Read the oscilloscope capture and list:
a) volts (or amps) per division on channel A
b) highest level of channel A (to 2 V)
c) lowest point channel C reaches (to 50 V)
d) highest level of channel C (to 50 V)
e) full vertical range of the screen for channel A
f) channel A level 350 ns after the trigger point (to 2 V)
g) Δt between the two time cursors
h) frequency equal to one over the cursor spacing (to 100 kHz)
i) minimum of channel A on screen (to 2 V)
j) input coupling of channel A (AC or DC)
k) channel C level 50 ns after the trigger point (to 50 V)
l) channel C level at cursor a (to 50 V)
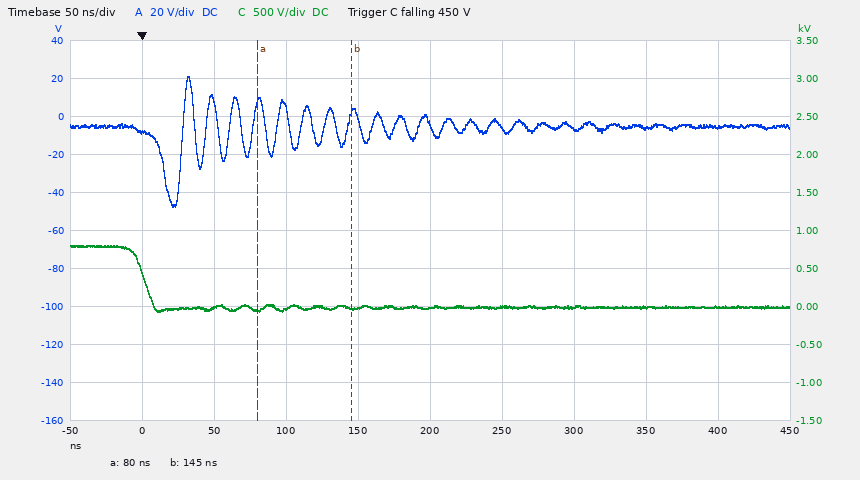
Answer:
20 V
22 V
-50 V
800 V
200 V
-6 V
65 ns
15.4 MHz
-48 V
DC
0 V
-50 V
